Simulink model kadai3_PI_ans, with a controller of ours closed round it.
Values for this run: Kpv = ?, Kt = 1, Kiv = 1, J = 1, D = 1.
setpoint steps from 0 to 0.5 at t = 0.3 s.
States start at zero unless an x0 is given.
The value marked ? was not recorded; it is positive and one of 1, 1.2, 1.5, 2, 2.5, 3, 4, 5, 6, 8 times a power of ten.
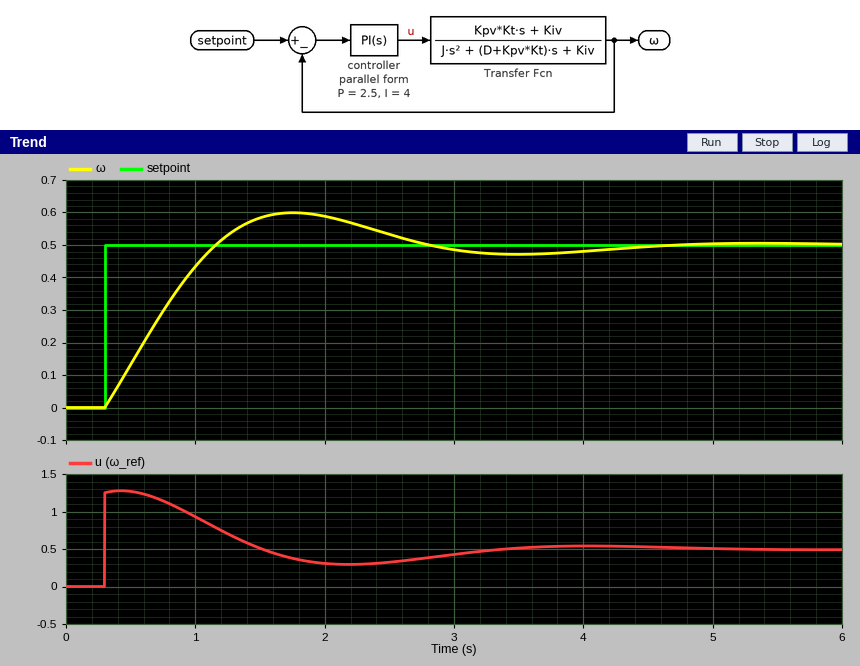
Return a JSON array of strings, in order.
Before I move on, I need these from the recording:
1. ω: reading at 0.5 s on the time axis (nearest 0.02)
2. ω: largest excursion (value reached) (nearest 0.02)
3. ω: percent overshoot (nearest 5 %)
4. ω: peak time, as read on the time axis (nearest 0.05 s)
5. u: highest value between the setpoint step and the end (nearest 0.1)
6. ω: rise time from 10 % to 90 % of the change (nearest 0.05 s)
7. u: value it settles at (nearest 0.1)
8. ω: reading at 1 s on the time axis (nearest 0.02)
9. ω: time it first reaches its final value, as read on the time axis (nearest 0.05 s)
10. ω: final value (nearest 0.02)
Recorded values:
["0.14", "0.60", "20 %", "1.75 s", "1.3", "0.65 s", "0.5", "0.44", "1.15 s", "0.50"]
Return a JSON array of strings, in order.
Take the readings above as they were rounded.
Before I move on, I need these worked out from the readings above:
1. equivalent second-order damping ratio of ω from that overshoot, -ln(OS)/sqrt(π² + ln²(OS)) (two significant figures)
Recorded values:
["0.46"]
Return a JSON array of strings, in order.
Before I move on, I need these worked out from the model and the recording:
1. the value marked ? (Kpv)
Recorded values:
["0.5"]
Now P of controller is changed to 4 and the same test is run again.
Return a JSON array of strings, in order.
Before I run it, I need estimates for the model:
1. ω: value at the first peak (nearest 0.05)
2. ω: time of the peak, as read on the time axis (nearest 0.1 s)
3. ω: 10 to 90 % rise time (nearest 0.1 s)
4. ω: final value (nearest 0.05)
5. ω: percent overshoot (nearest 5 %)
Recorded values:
["0.55", "1.5 s", "0.6 s", "0.50", "10 %"]
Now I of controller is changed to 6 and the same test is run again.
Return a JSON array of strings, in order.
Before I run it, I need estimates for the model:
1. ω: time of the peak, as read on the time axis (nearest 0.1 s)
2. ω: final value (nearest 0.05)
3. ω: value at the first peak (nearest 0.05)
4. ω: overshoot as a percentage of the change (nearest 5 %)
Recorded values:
["1.6 s", "0.50", "0.65", "30 %"]
